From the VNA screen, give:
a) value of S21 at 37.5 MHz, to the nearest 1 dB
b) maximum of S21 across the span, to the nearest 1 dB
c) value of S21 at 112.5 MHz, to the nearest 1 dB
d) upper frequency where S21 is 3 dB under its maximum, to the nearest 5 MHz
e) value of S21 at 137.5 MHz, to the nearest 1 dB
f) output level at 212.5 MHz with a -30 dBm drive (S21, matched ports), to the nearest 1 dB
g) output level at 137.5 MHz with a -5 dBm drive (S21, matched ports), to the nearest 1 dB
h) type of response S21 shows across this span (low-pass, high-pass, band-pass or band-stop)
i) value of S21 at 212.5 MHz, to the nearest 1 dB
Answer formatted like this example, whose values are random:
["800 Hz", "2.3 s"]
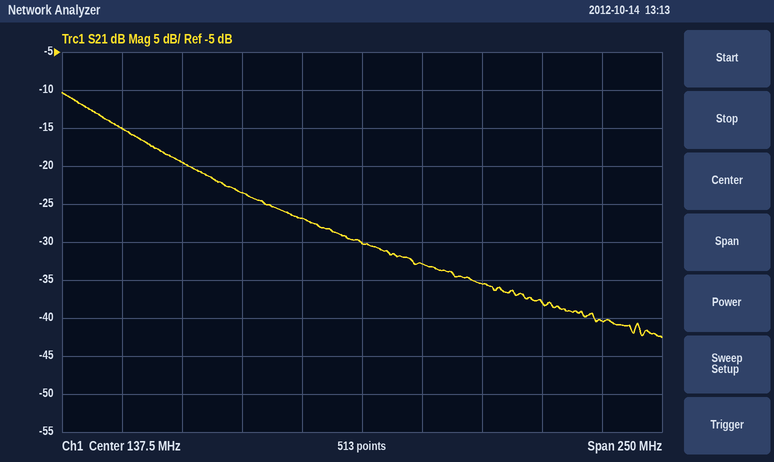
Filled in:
["-15 dB", "-10 dB", "-27 dB", "30 MHz", "-30 dB", "-68 dBm", "-35 dBm", "low-pass", "-38 dB"]
